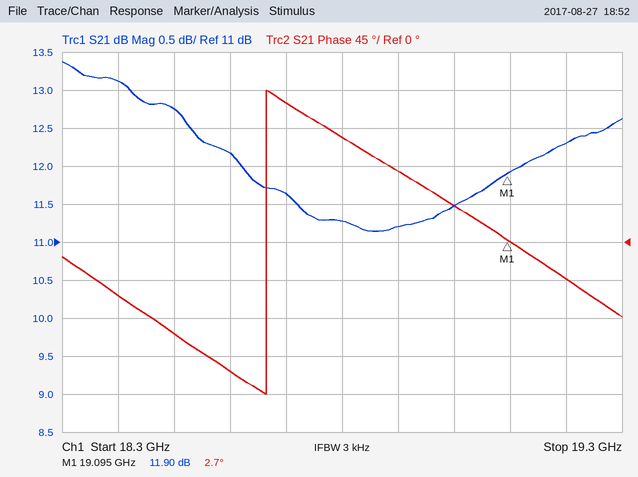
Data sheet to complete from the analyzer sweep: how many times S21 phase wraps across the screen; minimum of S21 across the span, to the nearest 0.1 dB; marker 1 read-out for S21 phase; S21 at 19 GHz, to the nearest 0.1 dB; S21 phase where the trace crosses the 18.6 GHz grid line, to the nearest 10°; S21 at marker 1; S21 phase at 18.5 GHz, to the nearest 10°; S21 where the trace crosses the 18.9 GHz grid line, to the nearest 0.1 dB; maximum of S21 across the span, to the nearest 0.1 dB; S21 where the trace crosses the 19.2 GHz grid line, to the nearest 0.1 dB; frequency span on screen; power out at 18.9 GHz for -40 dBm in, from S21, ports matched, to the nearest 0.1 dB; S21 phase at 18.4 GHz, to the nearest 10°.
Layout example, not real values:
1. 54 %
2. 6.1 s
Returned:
1. 1
2. 11.1 dB
3. 2.7°
4. 11.5 dB
5. -150°
6. 11.90 dB
7. -110°
8. 11.2 dB
9. 13.4 dB
10. 12.3 dB
11. 1 GHz
12. -28.8 dBm
13. -60°
